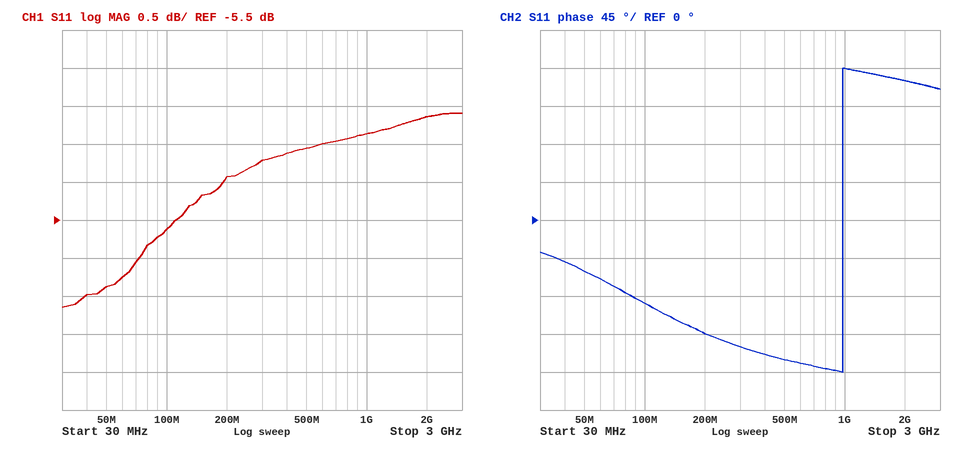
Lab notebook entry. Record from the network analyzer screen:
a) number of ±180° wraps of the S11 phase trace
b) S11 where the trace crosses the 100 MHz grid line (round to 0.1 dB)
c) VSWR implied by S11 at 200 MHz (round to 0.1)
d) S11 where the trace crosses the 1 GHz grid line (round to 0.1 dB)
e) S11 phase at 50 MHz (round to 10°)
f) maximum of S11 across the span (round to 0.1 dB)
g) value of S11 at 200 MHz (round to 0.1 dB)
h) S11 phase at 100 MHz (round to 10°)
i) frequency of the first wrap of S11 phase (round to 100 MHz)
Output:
1
-5.6 dB
3.6
-4.4 dB
-60°
-4.1 dB
-4.9 dB
-100°
1.0 GHz
